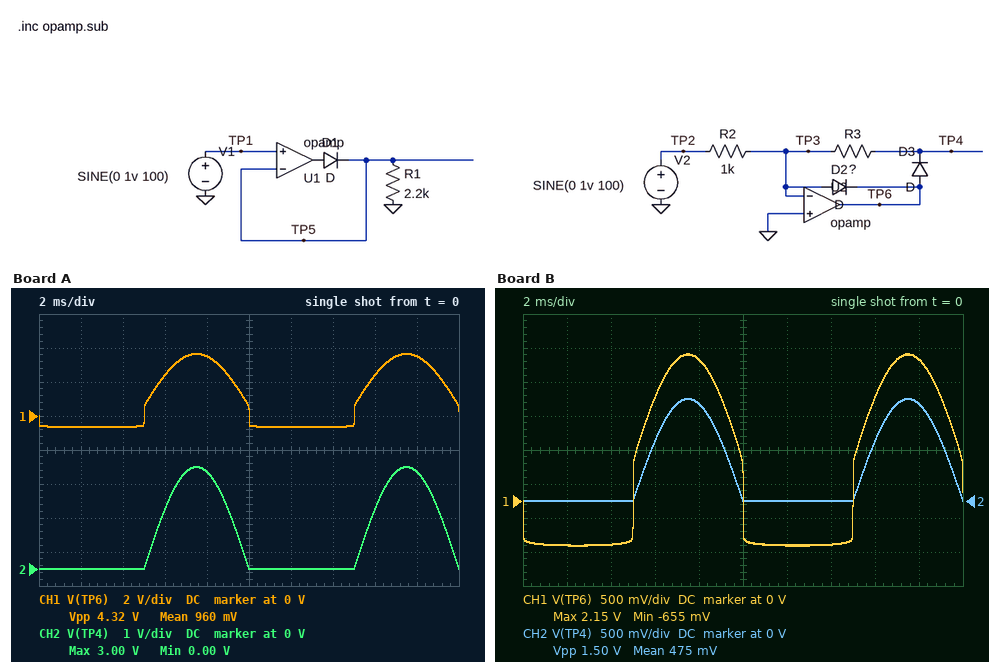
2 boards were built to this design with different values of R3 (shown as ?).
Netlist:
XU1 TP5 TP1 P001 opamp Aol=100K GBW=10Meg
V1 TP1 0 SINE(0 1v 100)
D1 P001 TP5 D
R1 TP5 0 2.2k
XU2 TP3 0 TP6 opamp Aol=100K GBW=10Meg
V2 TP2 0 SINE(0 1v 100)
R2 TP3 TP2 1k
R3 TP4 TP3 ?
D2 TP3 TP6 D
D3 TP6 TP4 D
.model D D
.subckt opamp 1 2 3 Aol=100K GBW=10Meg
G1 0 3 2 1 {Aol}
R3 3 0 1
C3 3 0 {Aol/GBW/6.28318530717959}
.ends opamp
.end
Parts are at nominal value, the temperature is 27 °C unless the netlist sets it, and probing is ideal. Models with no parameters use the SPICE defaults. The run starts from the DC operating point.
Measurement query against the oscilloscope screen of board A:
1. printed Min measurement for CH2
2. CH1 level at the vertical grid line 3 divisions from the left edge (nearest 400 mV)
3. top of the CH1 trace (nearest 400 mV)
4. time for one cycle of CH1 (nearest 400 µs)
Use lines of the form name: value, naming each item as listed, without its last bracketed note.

printed Min measurement for CH2: 0.00 V
CH1 level at the vertical grid line 3 divisions from the left edge: 2.4 V
top of the CH1 trace: 3.6 V
time for one cycle of CH1: 10.0 ms
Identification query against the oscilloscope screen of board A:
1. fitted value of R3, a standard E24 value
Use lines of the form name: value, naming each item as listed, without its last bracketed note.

fitted value of R3, a standard E24 value: 3 kΩ
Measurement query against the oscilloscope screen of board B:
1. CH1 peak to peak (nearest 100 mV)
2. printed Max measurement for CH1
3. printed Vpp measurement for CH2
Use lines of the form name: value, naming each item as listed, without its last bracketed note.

CH1 peak to peak: 2.8 V
printed Max measurement for CH1: 2.15 V
printed Vpp measurement for CH2: 1.50 V
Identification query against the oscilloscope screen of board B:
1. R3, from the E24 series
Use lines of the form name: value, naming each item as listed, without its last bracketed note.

R3, from the E24 series: 1.5 kΩ
